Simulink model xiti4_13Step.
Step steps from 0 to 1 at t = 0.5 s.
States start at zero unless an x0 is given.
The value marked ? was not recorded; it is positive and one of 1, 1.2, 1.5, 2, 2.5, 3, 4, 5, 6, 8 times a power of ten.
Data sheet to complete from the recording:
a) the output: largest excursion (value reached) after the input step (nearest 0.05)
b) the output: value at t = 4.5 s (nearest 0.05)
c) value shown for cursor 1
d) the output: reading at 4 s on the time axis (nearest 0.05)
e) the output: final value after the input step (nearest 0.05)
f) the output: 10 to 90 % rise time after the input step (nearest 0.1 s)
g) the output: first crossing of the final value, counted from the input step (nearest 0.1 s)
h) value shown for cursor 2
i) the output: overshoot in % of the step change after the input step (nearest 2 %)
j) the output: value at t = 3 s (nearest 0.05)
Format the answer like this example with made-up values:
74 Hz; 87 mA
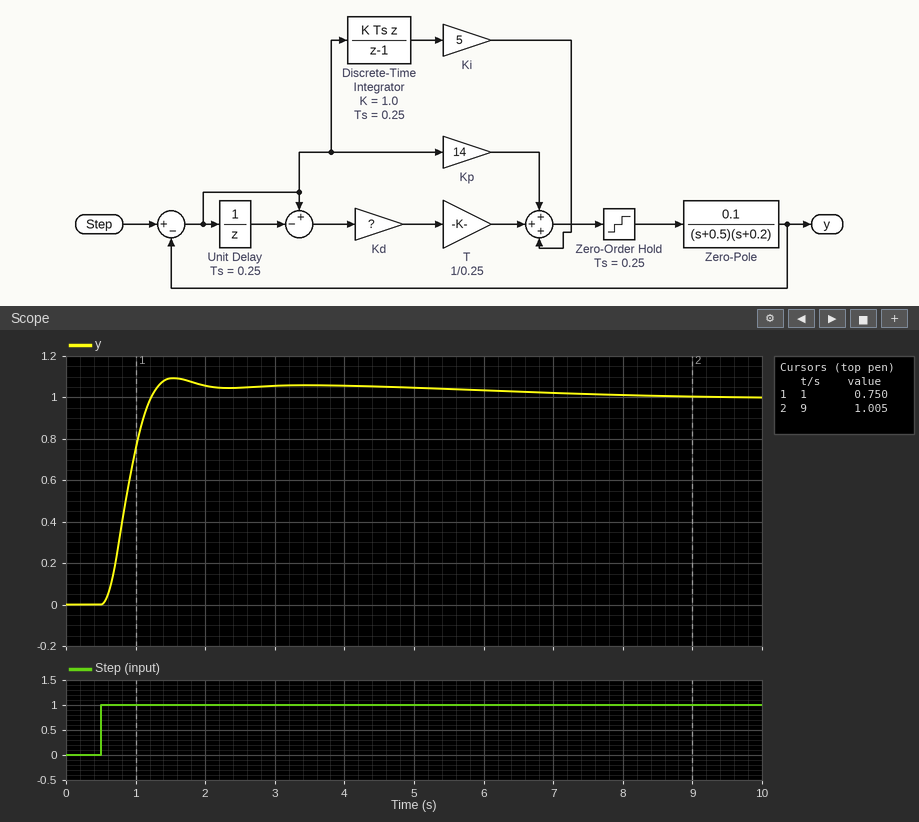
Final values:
1.10; 1.05; 0.750; 1.05; 1.00; 0.5 s; 0.7 s; 1.005; 10 %; 1.05
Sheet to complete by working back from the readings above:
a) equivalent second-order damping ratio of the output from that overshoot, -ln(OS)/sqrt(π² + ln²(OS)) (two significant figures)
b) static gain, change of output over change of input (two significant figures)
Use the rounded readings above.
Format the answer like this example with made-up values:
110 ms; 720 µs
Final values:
0.59; 1.0
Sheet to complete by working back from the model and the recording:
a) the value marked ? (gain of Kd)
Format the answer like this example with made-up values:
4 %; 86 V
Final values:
20
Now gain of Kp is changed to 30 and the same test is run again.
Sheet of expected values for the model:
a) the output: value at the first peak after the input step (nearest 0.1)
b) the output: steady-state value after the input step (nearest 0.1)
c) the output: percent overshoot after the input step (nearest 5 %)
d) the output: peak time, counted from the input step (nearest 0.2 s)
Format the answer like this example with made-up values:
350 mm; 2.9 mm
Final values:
1.3; 1.0; 30 %; 1.0 s
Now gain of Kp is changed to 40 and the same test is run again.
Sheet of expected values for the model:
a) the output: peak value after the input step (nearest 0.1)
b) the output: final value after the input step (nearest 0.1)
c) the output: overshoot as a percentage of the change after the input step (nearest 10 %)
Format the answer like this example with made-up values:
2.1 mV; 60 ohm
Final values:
1.4; 1.0; 40 %
